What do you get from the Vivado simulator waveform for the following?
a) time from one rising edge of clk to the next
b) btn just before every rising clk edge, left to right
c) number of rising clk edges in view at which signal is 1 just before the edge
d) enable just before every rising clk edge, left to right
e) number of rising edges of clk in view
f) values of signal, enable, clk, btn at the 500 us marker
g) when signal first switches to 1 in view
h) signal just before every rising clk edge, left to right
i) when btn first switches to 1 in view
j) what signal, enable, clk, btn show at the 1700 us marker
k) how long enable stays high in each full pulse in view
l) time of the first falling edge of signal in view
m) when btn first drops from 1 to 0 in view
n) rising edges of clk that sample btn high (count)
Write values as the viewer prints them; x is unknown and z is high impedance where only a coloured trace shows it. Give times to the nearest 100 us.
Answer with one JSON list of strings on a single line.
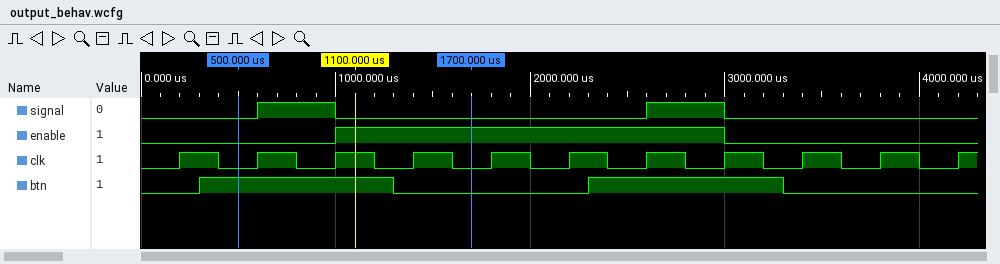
["400 us", "0 1 1 0 0 0 1 1 0 0 0", "2", "0 0 0 1 1 1 1 1 0 0 0", "11", "signal=0, enable=0, clk=0, btn=1", "600 us", "0 0 1 0 0 0 0 1 0 0 0", "300 us", "signal=0, enable=1, clk=0, btn=0", "2000 us", "1000 us", "1300 us", "4"]
